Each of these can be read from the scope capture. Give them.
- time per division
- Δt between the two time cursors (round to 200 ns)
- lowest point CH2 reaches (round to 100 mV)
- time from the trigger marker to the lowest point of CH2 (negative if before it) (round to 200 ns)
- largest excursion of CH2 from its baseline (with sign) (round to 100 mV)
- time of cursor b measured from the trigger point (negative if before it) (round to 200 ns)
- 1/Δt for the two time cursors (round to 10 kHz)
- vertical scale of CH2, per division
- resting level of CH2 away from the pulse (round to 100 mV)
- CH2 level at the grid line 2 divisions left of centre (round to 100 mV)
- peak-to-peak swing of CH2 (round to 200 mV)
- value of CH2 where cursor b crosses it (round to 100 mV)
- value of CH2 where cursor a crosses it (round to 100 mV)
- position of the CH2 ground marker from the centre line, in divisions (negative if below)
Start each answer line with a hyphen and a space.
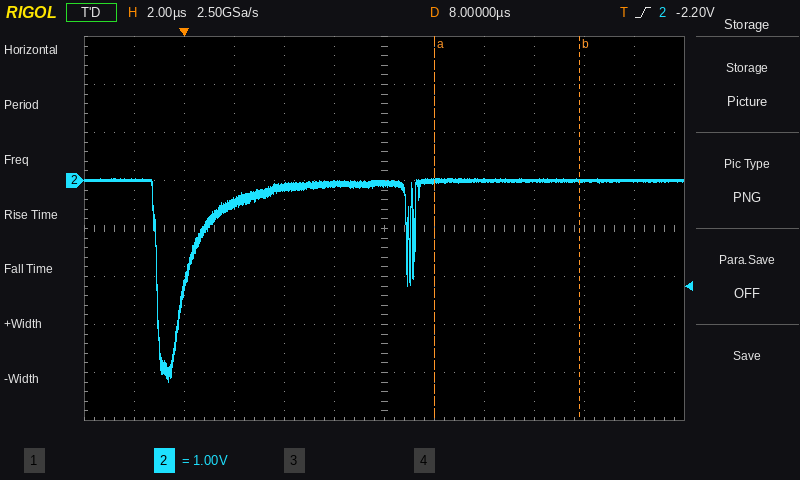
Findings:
- 2 µs
- 5.8 µs
- -4.2 V
- -600 ns
- -4.2 V
- +15.8 µs
- 170 kHz
- 1 V
- 0.0 V
- -100 mV
- 4.2 V
- 0.0 V
- 0.0 V
- +1.0 div
